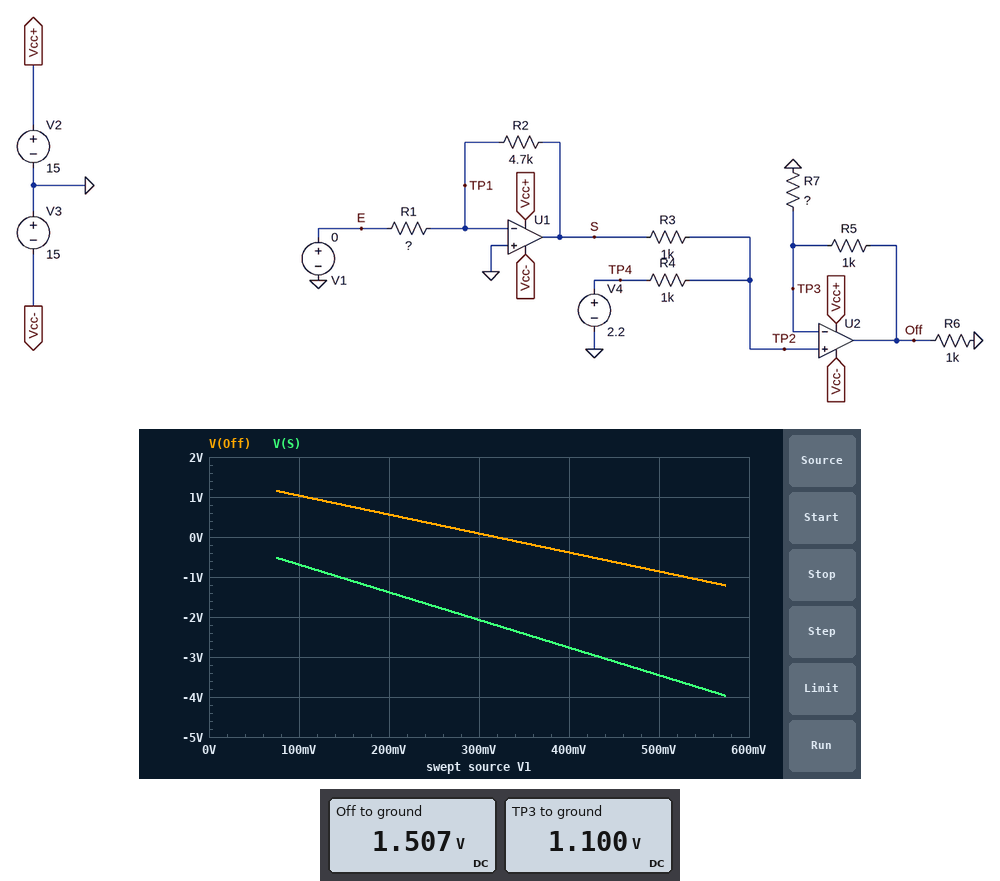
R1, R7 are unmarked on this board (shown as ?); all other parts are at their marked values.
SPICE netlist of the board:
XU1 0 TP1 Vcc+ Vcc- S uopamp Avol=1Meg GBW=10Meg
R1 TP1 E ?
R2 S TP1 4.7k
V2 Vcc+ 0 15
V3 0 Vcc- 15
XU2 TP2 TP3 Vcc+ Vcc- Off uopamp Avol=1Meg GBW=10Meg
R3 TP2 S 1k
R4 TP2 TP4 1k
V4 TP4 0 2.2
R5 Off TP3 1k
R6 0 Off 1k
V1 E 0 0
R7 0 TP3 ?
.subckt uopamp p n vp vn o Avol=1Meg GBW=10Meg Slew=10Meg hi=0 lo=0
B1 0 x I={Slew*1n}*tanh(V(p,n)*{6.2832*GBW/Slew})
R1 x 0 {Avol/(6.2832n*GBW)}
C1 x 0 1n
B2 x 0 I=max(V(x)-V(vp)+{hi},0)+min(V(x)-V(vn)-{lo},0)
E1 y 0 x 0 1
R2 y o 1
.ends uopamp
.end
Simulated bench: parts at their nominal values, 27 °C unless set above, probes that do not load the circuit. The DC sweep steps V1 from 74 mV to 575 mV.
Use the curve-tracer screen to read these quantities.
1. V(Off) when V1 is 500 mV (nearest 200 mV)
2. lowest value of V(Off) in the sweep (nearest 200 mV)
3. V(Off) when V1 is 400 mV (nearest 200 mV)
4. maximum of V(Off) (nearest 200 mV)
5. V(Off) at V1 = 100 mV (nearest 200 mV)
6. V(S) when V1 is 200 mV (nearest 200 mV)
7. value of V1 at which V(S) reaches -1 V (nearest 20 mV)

-800 mV
-1.2 V
-400 mV
1.2 V
1.0 V
-1.4 V
140 mV
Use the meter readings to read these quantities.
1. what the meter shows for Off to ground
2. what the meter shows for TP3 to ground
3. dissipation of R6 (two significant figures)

1.507 V
1.100 V
2.3 mW
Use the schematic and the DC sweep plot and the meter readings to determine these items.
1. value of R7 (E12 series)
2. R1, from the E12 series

2.7 kΩ
680 Ω
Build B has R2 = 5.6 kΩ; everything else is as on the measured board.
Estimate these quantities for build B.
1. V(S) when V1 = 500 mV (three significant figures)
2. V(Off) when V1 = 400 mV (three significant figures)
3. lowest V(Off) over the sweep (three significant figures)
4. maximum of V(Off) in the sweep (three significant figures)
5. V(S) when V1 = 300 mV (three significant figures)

-4.12 V
-750 mV
-1.74 V
1.09 V
-2.47 V
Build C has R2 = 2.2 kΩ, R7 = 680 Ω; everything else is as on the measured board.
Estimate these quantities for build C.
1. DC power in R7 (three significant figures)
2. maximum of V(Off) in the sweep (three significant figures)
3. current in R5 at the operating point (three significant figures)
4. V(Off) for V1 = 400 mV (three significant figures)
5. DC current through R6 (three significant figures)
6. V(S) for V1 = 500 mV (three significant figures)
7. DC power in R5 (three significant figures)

1.78 mW
2.42 V
1.62 mA
1.12 V
2.72 mA
-1.62 V
2.62 mW
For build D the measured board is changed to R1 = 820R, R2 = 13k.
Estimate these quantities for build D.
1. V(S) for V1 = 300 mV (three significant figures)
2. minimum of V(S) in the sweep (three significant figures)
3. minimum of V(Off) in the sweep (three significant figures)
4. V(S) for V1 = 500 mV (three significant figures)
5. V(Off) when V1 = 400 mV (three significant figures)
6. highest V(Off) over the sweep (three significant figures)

-4.76 V
-9.12 V
-4.74 V
-7.93 V
-2.84 V
704 mV
